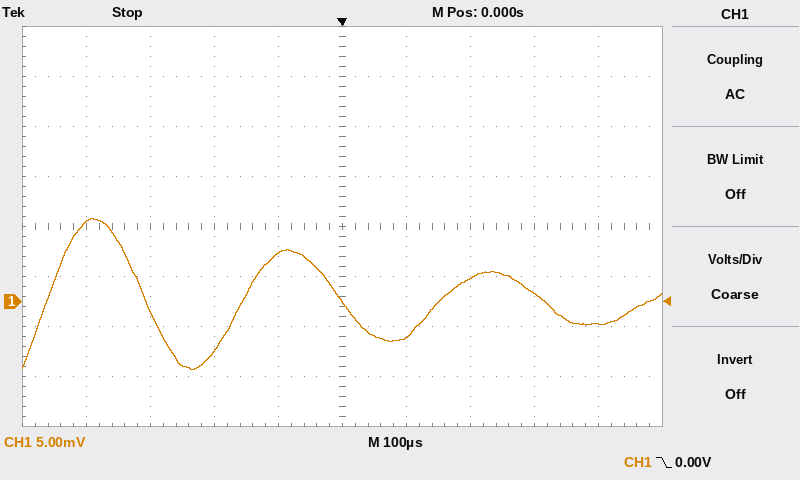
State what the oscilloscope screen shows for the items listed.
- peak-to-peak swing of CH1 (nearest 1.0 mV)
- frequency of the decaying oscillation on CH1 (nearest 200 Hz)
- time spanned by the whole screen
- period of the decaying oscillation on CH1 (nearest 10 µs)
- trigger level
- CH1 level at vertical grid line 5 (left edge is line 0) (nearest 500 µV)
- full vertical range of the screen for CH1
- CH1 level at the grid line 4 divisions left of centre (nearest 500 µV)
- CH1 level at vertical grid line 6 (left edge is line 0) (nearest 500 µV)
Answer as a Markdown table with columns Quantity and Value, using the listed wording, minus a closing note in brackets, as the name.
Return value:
| Quantity | Value |
|---|---|
| peak-to-peak swing of CH1 | 15.0 mV |
| frequency of the decaying oscillation on CH1 | 3.2 kHz |
| time spanned by the whole screen | 1 ms |
| period of the decaying oscillation on CH1 | 310 µs |
| trigger level | 0.00 V |
| CH1 level at vertical grid line 5 (left edge is line 0) | 0.0 mV |
| full vertical range of the screen for CH1 | 40 mV |
| CH1 level at the grid line 4 divisions left of centre | 8.0 mV |
| CH1 level at vertical grid line 6 (left edge is line 0) | -3.5 mV |
